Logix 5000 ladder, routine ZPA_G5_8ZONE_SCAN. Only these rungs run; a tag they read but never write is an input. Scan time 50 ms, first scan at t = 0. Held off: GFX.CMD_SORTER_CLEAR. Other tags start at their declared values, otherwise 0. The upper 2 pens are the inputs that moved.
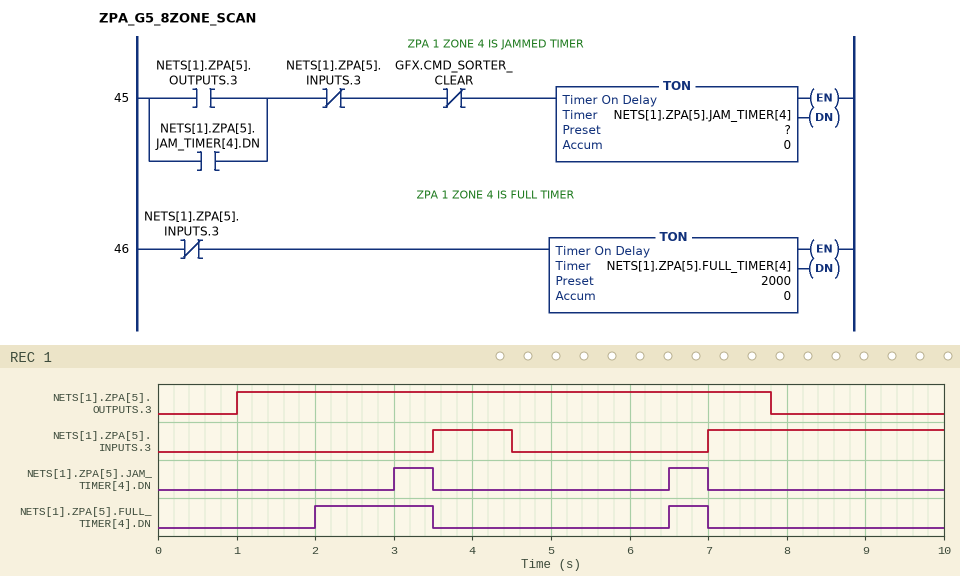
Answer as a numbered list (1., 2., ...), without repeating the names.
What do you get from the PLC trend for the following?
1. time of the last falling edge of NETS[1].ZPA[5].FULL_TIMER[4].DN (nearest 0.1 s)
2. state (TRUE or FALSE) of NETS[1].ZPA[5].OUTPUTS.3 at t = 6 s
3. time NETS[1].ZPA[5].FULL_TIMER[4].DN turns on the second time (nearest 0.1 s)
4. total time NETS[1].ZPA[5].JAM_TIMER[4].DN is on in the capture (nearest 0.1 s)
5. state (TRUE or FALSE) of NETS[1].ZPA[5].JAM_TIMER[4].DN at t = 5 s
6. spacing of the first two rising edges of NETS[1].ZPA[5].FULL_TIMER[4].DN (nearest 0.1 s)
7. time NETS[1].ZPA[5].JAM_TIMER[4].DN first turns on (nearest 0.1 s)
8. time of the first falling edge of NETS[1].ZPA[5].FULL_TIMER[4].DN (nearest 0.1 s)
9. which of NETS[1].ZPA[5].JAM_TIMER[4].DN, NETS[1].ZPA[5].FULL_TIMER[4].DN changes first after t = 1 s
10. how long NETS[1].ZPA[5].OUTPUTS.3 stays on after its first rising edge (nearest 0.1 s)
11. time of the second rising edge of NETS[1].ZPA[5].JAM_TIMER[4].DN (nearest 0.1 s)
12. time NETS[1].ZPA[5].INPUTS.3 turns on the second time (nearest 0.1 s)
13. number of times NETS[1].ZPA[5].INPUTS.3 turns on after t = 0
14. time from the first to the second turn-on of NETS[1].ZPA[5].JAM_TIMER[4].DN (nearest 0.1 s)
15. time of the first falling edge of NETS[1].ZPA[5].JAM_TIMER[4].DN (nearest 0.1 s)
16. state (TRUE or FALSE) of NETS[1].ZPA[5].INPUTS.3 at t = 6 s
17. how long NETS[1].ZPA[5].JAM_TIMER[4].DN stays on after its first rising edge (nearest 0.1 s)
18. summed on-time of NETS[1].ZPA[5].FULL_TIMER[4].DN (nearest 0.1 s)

1. 7.0 s
2. TRUE
3. 6.5 s
4. 1.0 s
5. FALSE
6. 4.5 s
7. 3.0 s
8. 3.5 s
9. NETS[1].ZPA[5].FULL_TIMER[4].DN
10. 6.8 s
11. 6.5 s
12. 7.0 s
13. 2
14. 3.5 s
15. 3.5 s
16. FALSE
17. 0.5 s
18. 2.0 s
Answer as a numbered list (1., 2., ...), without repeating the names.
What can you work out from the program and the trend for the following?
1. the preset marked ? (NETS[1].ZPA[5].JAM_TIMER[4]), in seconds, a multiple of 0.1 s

1. 2.0 s
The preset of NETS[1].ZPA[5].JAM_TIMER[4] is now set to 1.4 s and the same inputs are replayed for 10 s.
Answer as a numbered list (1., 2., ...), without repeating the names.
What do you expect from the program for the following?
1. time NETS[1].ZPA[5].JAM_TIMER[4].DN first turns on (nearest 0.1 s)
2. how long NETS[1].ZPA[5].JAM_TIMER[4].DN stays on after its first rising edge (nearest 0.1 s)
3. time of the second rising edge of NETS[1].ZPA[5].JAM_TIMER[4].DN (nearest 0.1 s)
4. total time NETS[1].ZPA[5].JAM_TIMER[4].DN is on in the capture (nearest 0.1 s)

1. 2.4 s
2. 1.1 s
3. 5.9 s
4. 2.2 s
